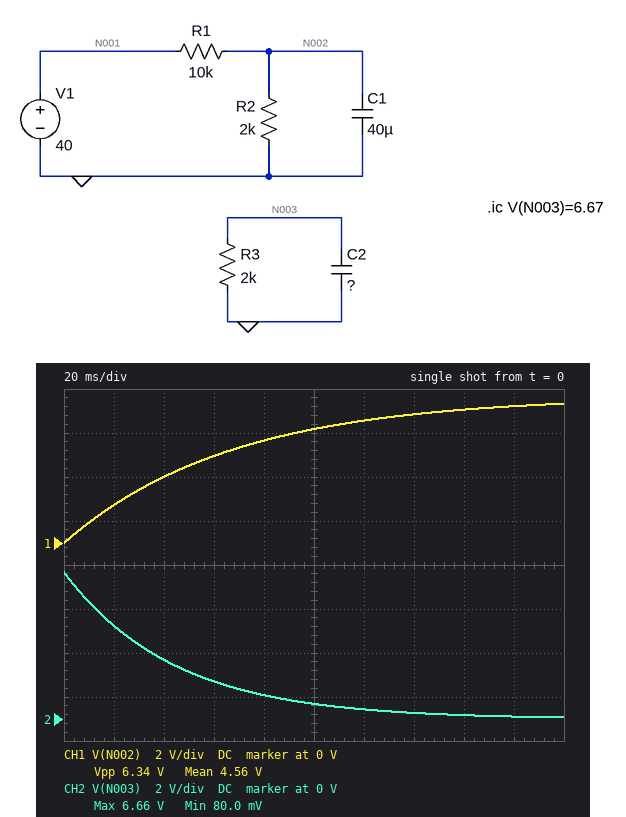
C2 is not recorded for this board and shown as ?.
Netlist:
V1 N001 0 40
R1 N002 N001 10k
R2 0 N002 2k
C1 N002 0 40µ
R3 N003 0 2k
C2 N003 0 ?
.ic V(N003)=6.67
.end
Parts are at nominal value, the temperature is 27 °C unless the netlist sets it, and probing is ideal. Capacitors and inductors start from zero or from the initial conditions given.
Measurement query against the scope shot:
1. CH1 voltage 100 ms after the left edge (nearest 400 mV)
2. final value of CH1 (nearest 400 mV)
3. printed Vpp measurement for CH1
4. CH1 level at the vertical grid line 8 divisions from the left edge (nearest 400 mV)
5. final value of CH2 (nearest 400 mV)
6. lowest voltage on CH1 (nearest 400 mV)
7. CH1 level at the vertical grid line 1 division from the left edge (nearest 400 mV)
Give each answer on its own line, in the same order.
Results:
5.2 V
6.4 V
6.34 V
6.0 V
0 V
0 V
1.6 V
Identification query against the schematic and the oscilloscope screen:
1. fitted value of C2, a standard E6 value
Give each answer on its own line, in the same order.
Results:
22 µF
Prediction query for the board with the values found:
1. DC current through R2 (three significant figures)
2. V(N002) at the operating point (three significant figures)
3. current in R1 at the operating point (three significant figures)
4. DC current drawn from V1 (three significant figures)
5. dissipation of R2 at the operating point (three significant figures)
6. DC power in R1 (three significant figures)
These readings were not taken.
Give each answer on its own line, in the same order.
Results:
3.33 mA
6.67 V
3.33 mA
3.33 mA
22.2 mW
111 mW
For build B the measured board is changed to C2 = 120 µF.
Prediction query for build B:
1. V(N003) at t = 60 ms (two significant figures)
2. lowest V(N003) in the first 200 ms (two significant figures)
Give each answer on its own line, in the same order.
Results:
5.2 V
2.9 V
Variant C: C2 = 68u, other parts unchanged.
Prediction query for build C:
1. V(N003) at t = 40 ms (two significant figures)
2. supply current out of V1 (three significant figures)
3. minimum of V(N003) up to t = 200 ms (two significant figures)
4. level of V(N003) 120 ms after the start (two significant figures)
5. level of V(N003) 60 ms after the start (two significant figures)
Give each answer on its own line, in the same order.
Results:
5.0 V
3.33 mA
1.5 V
2.8 V
4.3 V
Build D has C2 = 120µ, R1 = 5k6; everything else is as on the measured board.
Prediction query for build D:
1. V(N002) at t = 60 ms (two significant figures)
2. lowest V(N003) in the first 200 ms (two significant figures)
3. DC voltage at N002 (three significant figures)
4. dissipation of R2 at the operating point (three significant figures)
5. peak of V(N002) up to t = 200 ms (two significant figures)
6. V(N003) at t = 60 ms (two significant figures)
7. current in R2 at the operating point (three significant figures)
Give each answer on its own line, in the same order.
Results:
6.7 V
2.9 V
10.5 V
55.4 mW
10 V
5.2 V
5.26 mA
